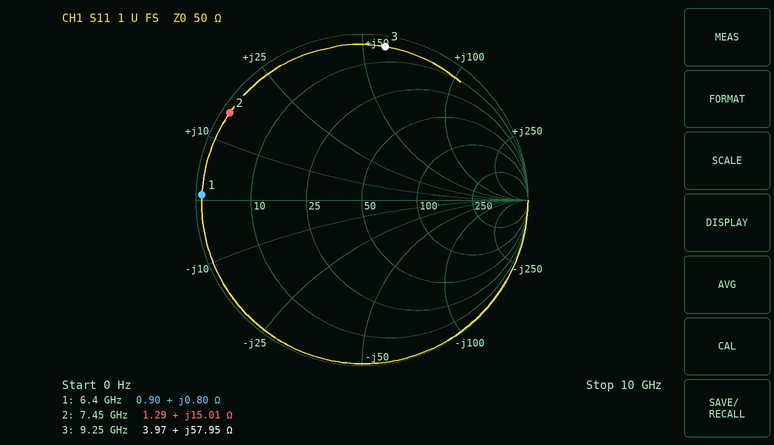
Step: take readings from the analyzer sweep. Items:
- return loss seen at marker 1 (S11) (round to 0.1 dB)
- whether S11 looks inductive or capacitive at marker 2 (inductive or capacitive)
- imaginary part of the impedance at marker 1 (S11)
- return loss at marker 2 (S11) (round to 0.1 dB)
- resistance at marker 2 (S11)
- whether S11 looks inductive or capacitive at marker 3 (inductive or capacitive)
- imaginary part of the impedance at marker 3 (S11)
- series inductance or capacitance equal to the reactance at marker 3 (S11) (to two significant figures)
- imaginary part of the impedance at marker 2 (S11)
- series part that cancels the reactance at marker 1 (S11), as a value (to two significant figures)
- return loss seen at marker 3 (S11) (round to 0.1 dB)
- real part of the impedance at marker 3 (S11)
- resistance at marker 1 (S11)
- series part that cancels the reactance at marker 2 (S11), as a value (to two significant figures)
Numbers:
0.3 dB
inductive
+0.80 Ω
0.4 dB
1.29 Ω
inductive
+57.95 Ω
1.00 nH
+15.01 Ω
31 pF
0.6 dB
3.97 Ω
0.90 Ω
1.4 pF
